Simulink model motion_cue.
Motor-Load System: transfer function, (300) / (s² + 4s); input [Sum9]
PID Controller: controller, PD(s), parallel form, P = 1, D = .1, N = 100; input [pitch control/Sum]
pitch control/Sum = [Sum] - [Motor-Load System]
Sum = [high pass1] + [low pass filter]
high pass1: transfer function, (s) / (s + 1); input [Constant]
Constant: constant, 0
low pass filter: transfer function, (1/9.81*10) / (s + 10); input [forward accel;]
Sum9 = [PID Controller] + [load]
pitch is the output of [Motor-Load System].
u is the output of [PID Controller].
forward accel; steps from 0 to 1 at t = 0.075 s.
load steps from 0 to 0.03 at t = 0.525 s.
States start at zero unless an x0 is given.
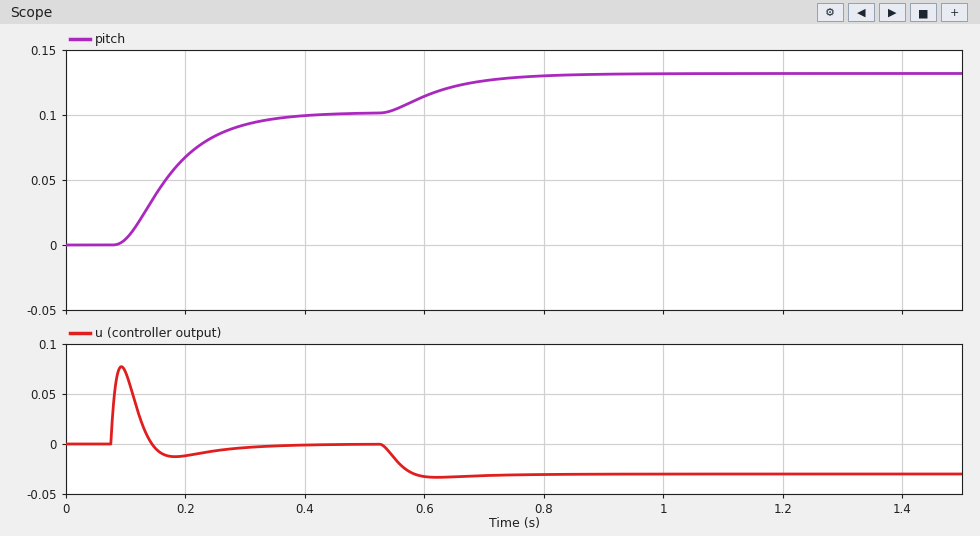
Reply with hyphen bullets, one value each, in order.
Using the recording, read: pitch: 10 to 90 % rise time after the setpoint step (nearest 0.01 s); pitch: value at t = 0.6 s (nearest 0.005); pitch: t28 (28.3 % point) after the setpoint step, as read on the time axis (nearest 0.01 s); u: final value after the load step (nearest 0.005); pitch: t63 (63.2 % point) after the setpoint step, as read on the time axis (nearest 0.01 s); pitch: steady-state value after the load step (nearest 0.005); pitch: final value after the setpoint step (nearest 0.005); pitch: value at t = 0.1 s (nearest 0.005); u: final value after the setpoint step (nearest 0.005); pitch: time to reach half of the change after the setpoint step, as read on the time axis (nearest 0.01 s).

- 0.18 s
- 0.115
- 0.14 s
- -0.030
- 0.19 s
- 0.130
- 0.100
- 0.005
- 0.000
- 0.17 s
